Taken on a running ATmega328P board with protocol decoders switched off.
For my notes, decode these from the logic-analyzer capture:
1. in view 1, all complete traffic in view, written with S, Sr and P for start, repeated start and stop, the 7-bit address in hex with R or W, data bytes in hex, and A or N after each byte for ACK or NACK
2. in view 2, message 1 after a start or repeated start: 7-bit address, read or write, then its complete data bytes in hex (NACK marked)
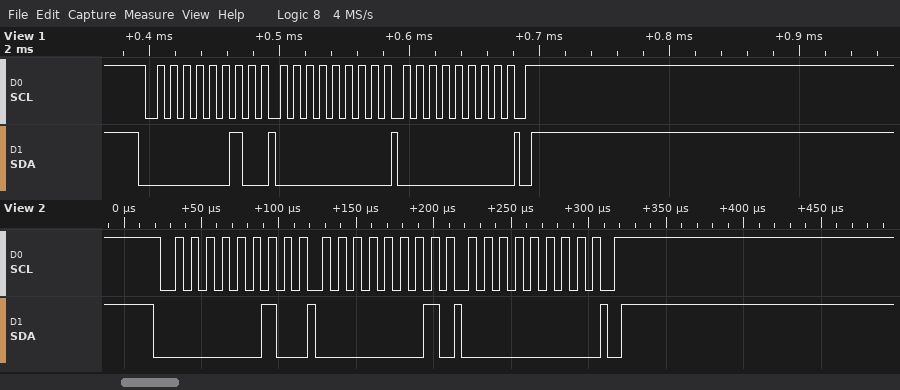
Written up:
S 01W A 00 A 00 A P
0x01 write: 01 00
